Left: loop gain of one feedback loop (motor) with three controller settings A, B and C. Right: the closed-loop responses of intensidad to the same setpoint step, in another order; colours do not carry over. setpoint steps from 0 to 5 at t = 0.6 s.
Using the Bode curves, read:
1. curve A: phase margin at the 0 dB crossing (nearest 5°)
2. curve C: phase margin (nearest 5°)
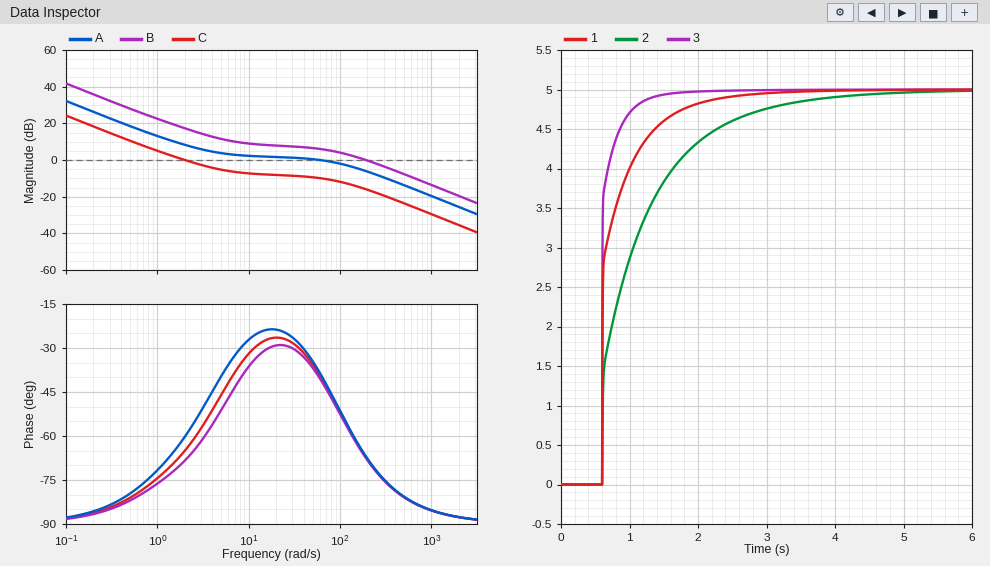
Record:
140°
115°
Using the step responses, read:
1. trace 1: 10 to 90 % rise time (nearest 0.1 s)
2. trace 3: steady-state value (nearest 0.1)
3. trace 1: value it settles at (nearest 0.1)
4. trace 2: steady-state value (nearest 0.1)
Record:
0.8 s
5.0
5.0
5.0
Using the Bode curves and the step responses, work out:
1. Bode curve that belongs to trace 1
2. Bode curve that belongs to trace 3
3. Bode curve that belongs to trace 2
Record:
A
B
C
